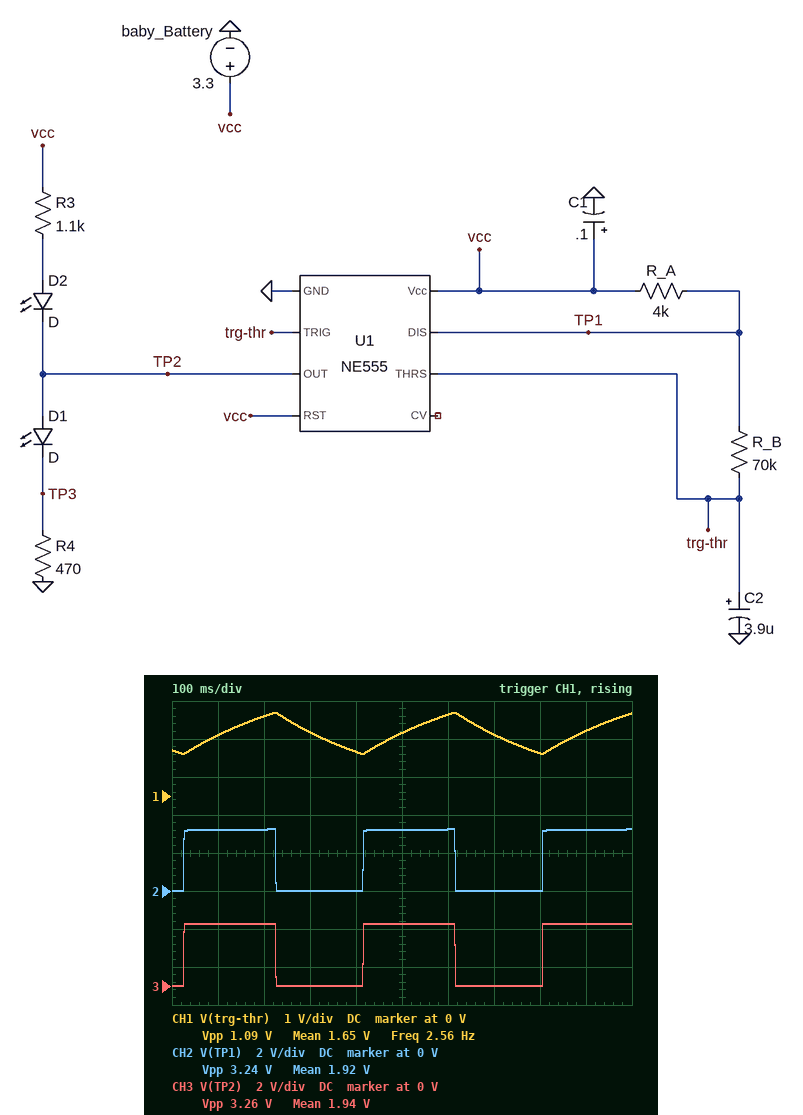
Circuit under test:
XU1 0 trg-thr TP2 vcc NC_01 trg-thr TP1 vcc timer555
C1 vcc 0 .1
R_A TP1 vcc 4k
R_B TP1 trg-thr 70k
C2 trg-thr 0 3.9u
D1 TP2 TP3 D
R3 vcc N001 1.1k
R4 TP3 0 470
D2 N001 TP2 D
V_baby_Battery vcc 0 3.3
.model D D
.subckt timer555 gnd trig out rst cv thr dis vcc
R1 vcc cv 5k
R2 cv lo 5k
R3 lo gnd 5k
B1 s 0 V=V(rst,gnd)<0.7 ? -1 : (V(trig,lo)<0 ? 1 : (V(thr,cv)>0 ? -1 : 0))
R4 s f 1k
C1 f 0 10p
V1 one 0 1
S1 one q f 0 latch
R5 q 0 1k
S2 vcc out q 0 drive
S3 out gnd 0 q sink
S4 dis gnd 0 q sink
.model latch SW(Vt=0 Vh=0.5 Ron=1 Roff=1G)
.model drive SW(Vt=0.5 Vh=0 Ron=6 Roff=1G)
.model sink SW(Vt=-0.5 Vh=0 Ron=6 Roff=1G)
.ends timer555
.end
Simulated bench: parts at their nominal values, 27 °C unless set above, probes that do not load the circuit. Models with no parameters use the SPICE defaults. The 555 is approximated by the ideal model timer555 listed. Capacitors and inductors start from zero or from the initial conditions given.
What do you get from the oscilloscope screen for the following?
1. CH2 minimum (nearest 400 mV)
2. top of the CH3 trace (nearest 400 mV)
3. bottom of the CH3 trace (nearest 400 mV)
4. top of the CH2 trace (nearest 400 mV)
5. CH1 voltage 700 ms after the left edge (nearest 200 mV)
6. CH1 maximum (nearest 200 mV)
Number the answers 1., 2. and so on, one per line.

1. 0 V
2. 3.2 V
3. 0 V
4. 3.2 V
5. 1.6 V
6. 2.2 V
